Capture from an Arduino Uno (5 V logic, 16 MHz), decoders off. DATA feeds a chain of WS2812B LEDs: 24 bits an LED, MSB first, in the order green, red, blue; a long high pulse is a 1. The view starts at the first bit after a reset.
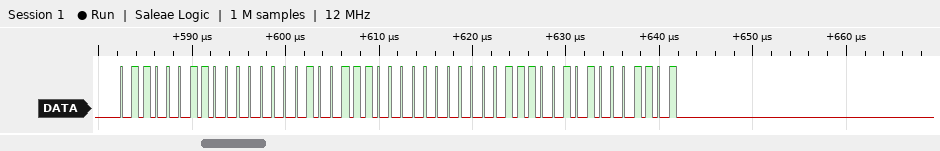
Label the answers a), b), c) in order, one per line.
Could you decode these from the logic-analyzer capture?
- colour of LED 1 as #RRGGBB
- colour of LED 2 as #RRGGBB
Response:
a) #00639C
b) #72008D
